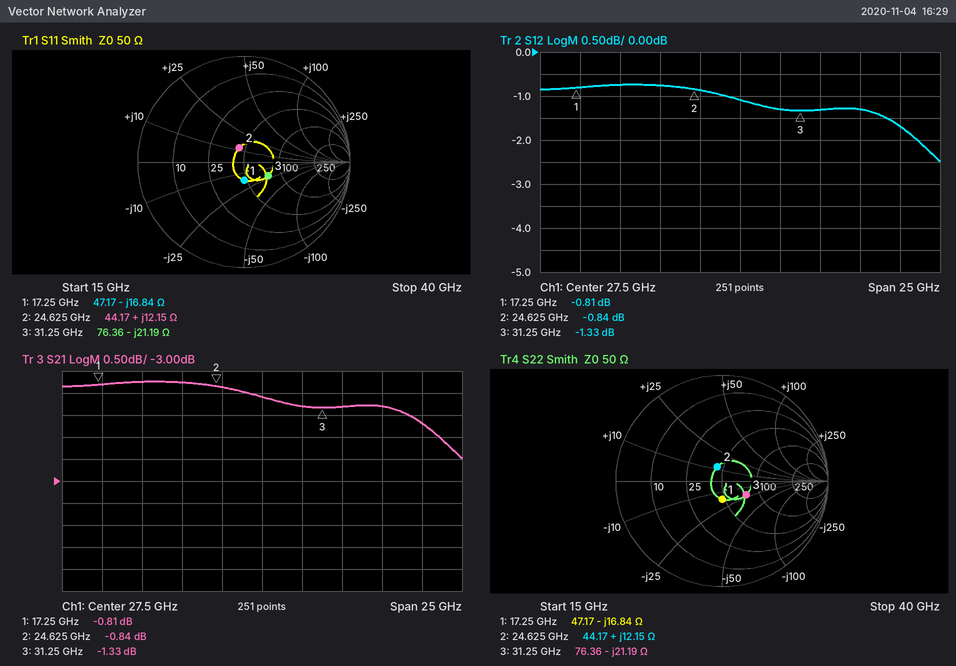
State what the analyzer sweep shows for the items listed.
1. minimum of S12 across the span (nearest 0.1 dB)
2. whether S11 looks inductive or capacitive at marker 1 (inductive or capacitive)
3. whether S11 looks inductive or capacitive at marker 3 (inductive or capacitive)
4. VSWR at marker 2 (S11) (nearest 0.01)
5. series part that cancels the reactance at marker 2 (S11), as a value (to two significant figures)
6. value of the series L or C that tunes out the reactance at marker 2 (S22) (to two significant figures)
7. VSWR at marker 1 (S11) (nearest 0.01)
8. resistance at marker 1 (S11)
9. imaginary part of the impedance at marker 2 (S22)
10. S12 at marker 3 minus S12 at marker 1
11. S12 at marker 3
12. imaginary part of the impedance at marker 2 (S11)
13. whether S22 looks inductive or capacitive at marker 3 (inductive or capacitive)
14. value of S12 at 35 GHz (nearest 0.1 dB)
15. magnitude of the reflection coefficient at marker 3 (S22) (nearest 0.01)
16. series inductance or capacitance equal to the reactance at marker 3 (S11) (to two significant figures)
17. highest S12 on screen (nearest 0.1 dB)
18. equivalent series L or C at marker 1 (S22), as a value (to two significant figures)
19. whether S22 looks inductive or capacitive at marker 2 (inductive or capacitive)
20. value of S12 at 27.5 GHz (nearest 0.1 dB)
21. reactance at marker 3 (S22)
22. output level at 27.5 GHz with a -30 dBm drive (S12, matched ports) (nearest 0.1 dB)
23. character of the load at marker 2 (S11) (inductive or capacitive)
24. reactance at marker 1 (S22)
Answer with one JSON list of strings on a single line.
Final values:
["-2.5 dB", "capacitive", "capacitive", "1.33", "530 fF", "530 fF", "1.42", "47.17 Ω", "+12.15 Ω", "-0.52 dB", "-1.33 dB", "+12.15 Ω", "capacitive", "-1.3 dB", "0.26", "240 fF", "-0.7 dB", "550 fF", "inductive", "-1.1 dB", "-21.19 Ω", "-31.1 dBm", "inductive", "-16.84 Ω"]
